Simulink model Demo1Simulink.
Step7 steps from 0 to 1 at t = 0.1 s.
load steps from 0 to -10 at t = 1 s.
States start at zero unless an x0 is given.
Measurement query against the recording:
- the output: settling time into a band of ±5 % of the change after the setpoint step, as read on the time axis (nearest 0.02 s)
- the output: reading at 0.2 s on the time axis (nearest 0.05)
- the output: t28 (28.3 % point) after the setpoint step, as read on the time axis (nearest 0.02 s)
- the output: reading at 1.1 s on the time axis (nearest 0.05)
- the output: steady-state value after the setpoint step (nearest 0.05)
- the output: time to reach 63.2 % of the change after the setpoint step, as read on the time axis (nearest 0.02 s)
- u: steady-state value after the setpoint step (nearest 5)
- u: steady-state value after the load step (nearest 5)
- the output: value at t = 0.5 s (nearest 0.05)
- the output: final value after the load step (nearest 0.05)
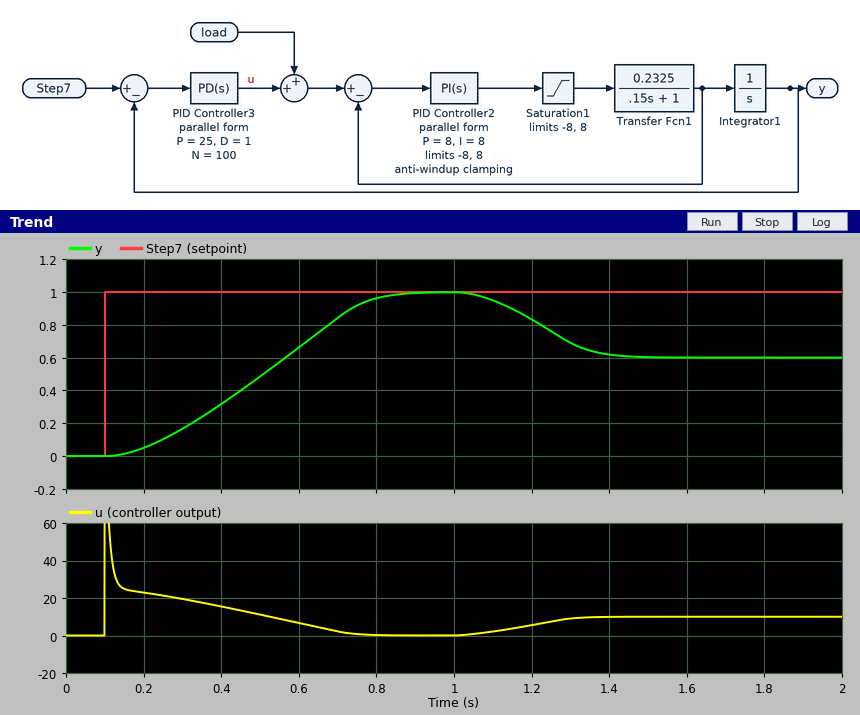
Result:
0.78 s
0.05
0.38 s
0.95
1.00
0.58 s
0
10
0.50
0.60
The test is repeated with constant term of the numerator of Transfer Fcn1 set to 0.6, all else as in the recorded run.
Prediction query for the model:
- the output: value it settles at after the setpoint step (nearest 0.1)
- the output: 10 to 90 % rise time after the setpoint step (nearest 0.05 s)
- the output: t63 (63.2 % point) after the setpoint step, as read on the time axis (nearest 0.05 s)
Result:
1.0
0.25 s
0.35 s
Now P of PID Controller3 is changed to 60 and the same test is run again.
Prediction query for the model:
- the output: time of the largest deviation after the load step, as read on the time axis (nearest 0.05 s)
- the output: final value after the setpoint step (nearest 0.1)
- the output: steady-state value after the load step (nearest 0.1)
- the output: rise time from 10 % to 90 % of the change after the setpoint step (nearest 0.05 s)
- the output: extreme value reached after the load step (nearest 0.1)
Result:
1.25 s
1.0
0.8
0.50 s
0.8
